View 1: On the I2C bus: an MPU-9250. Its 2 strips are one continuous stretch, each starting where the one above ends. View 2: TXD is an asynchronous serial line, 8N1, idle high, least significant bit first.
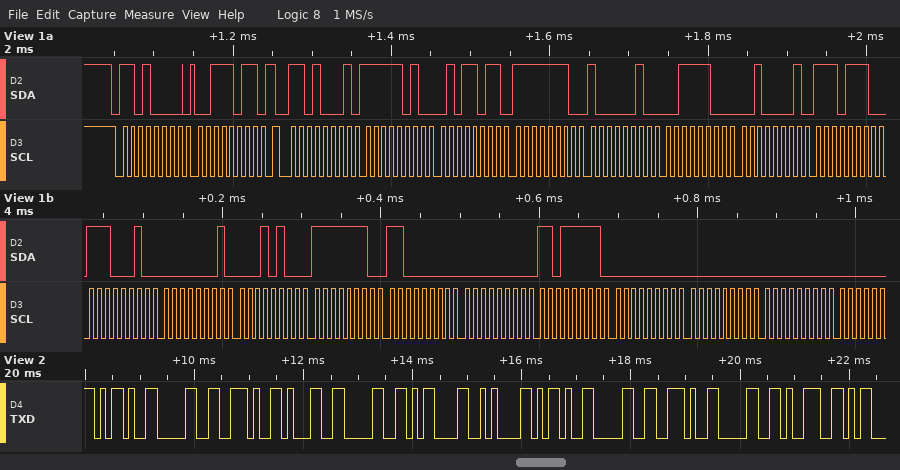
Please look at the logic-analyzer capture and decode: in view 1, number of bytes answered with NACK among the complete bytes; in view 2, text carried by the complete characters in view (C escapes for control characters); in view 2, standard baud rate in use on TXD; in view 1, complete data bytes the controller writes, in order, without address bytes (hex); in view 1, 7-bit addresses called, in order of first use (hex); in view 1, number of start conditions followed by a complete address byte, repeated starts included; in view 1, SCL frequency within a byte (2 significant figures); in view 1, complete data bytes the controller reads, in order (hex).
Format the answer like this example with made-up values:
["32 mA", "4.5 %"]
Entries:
["0", "\"-0.10\\r\\n-0.09\"", "9600 baud", "3B", "0x68", "2", "100 kHz", "FA 5B FE 82 3C 21 EE E2 01 14 FE C0 00 DF 00 00 00"]
